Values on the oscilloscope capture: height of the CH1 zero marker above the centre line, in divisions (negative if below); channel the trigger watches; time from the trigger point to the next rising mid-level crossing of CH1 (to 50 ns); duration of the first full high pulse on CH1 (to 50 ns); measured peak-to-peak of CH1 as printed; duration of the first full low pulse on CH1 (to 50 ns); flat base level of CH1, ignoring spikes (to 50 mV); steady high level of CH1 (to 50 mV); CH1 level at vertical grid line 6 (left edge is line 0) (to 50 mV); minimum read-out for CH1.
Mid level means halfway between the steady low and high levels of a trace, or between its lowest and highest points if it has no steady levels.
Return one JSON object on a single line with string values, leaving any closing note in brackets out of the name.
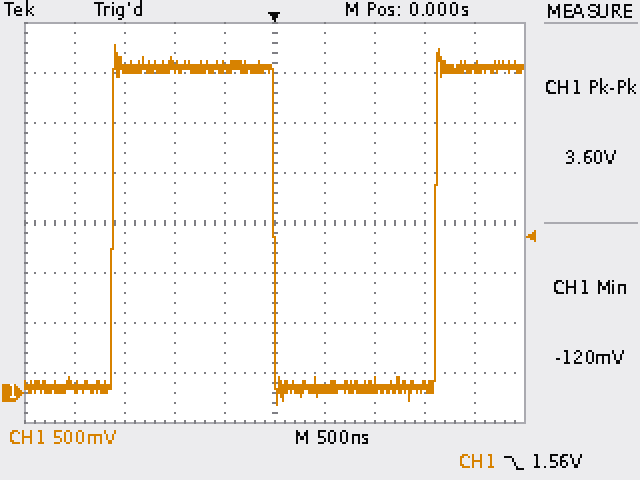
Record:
{"height of the CH1 zero marker above the centre line, in divisions": "-3.4 div", "channel the trigger watches": "CH1", "time from the trigger point to the next rising mid-level crossing of CH1": "1.60 µs", "duration of the first full high pulse on CH1": "1.60 µs", "measured peak-to-peak of CH1 as printed": "3.60 V", "duration of the first full low pulse on CH1": "1.60 µs", "flat base level of CH1, ignoring spikes": "50 mV", "steady high level of CH1": "3.25 V", "CH1 level at vertical grid line 6 (left edge is line 0)": "50 mV", "minimum read-out for CH1": "-120 mV"}
